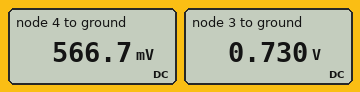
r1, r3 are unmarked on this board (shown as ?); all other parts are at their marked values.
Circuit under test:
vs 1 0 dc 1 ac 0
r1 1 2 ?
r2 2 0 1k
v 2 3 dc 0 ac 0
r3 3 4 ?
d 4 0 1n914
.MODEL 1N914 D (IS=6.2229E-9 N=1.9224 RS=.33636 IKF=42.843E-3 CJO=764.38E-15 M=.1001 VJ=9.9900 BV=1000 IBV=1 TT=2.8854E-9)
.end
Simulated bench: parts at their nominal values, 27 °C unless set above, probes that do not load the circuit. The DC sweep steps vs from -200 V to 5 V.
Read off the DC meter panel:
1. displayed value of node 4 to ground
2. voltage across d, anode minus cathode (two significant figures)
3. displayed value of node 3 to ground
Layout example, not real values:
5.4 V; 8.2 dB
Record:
566.7 mV; 570 mV; 0.730 V
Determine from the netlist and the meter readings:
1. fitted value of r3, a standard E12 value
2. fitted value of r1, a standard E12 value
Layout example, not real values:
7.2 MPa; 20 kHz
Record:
330 Ω; 220 Ω
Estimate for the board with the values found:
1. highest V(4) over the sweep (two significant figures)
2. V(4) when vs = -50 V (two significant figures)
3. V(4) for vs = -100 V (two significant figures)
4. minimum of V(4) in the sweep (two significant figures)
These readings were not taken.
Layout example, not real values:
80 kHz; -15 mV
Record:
710 mV; -41 V; -82 V; -160 V
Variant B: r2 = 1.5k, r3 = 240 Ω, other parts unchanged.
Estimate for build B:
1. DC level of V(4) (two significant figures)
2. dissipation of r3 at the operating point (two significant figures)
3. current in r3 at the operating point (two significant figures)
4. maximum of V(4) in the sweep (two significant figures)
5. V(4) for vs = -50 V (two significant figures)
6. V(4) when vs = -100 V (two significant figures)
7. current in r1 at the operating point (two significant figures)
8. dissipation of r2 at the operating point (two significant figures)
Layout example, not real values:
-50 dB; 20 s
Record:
580 mV; 110 µW; 670 µA; 730 mV; -44 V; -87 V; 1.2 mA; 370 µW
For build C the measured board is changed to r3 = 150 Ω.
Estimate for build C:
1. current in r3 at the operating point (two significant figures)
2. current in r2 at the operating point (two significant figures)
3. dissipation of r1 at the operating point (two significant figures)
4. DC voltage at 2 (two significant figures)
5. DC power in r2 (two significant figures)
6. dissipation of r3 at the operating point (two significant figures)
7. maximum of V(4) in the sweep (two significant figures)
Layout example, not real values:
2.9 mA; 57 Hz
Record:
710 µA; 690 µA; 430 µW; 690 mV; 480 µW; 75 µW; 740 mV
